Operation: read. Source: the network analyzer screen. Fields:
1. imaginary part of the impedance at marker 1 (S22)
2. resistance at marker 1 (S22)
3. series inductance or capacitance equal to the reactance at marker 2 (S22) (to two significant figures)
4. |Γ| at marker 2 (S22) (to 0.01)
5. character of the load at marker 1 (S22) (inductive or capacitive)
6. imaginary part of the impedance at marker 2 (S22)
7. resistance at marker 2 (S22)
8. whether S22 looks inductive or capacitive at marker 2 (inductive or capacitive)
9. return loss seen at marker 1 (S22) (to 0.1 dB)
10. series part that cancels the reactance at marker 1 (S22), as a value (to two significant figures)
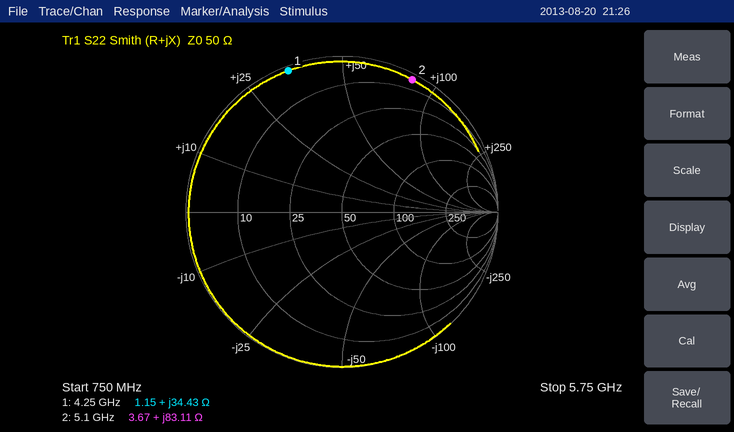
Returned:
+34.43 Ω
1.15 Ω
2.6 nH
0.96
inductive
+83.11 Ω
3.67 Ω
inductive
0.3 dB
1.1 pF
